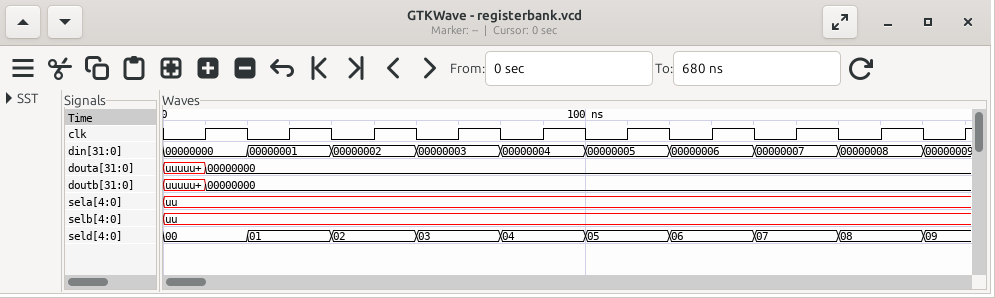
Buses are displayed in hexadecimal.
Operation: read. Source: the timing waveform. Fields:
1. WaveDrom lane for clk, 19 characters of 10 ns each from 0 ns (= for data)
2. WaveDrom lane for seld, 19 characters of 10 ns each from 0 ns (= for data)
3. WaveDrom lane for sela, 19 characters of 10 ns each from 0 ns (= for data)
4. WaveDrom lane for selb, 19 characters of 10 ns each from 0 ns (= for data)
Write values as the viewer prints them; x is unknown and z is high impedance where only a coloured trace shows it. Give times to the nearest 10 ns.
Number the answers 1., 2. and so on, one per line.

1. {name: 'clk', wave: '0101010101010101010'}
2. {name: 'seld', wave: '=.=.=.=.=.=.=.=.=.=', data: '00 01 02 03 04 05 06 07 08 09'}
3. {name: 'sela', wave: 'x..................'}
4. {name: 'selb', wave: 'x..................'}
